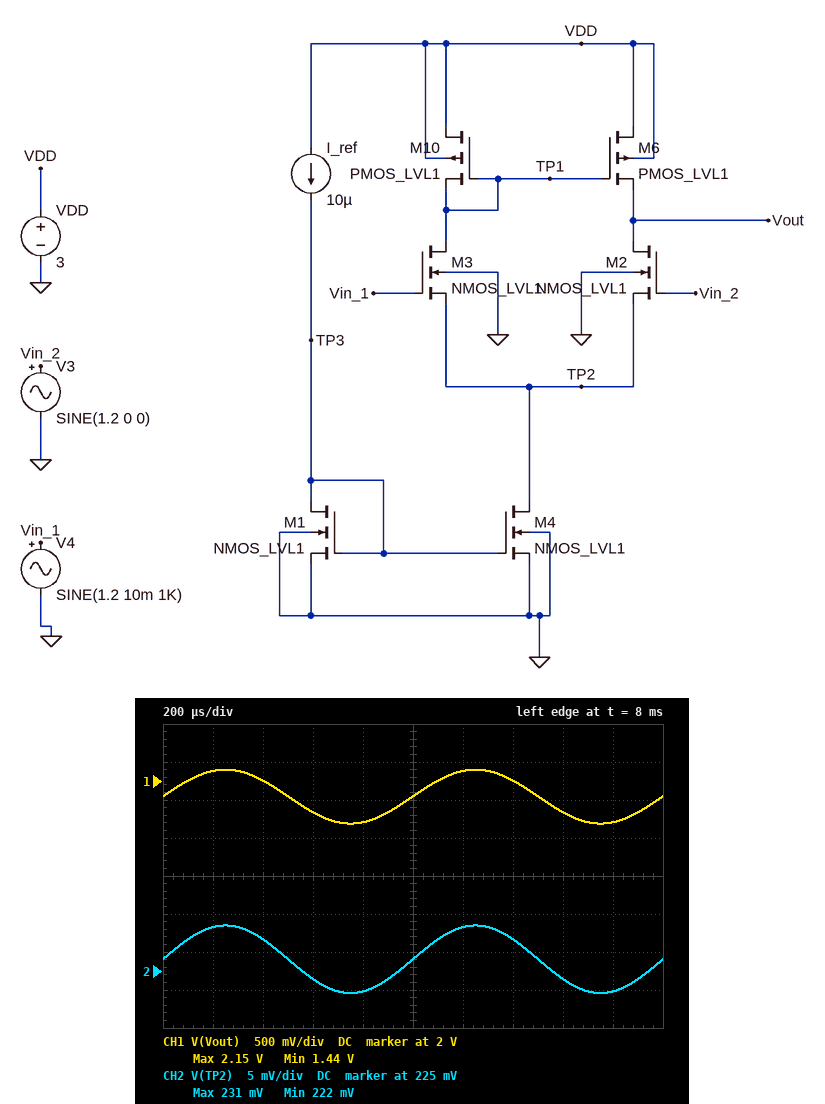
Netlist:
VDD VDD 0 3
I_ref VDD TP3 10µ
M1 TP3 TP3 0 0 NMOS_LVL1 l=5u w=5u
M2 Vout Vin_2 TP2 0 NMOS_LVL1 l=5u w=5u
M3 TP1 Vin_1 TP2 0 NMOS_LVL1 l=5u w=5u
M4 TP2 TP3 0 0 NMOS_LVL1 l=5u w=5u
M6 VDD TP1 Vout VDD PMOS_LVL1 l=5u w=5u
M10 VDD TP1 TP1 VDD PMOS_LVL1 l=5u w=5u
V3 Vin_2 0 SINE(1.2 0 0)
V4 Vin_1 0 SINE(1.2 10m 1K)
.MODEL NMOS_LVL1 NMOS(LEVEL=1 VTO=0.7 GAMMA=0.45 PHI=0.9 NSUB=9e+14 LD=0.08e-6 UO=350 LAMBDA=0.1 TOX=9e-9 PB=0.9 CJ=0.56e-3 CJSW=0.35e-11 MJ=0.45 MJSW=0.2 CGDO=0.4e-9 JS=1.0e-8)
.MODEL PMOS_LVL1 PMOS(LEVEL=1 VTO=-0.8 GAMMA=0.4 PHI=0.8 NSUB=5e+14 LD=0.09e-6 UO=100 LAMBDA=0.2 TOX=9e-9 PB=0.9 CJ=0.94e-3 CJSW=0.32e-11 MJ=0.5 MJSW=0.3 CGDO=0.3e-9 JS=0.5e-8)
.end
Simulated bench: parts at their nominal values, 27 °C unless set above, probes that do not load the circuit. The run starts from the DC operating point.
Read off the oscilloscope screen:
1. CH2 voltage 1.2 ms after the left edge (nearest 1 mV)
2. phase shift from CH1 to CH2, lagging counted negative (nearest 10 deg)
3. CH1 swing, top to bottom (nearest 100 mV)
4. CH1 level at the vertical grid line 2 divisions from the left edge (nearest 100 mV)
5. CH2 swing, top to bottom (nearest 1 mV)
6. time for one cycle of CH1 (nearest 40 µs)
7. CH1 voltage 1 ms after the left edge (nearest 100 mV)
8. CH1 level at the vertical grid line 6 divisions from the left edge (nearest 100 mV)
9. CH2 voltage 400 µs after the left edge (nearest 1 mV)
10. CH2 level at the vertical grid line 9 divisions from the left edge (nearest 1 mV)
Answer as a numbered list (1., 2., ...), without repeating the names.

1. 231 mV
2. 0 deg
3. 700 mV
4. 2.0 V
5. 9 mV
6. 1.00 ms
7. 1.8 V
8. 2.1 V
9. 229 mV
10. 222 mV
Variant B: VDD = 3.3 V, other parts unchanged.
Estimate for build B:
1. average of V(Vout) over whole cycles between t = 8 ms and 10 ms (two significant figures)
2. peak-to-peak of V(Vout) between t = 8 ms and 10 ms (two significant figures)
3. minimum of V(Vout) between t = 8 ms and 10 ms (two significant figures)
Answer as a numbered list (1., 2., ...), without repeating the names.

1. 2.1 V
2. 720 mV
3. 1.7 V
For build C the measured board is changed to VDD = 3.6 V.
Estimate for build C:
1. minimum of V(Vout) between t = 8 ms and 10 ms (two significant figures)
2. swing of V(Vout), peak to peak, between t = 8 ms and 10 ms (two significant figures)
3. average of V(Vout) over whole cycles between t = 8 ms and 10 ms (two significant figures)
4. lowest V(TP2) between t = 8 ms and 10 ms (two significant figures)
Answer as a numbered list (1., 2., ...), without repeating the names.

1. 2.0 V
2. 740 mV
3. 2.4 V
4. 230 mV
